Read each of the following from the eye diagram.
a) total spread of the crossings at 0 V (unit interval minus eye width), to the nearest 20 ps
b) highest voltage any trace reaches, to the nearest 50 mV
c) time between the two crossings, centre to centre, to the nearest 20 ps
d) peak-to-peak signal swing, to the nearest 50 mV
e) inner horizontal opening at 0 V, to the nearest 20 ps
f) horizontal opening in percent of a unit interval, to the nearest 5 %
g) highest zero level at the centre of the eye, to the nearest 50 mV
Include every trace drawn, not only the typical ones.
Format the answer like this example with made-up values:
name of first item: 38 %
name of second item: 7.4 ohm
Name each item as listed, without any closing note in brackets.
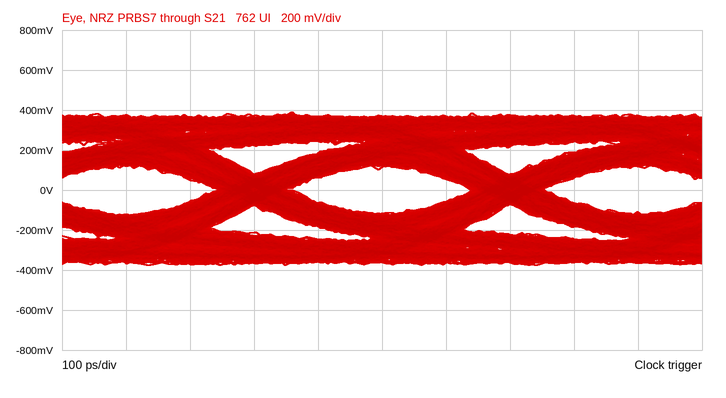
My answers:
total spread of the crossings at 0 V (unit interval minus eye width), to the nearest 20 ps: 120 ps
highest voltage any trace reaches, to the nearest 50 mV: 400 mV
time between the two crossings, centre to centre, to the nearest 20 ps: 400 ps
peak-to-peak signal swing, to the nearest 50 mV: 750 mV
inner horizontal opening at 0 V, to the nearest 20 ps: 280 ps
horizontal opening in percent of a unit interval, to the nearest 5 %: 70 %
highest zero level at the centre of the eye, to the nearest 50 mV: -100 mV
